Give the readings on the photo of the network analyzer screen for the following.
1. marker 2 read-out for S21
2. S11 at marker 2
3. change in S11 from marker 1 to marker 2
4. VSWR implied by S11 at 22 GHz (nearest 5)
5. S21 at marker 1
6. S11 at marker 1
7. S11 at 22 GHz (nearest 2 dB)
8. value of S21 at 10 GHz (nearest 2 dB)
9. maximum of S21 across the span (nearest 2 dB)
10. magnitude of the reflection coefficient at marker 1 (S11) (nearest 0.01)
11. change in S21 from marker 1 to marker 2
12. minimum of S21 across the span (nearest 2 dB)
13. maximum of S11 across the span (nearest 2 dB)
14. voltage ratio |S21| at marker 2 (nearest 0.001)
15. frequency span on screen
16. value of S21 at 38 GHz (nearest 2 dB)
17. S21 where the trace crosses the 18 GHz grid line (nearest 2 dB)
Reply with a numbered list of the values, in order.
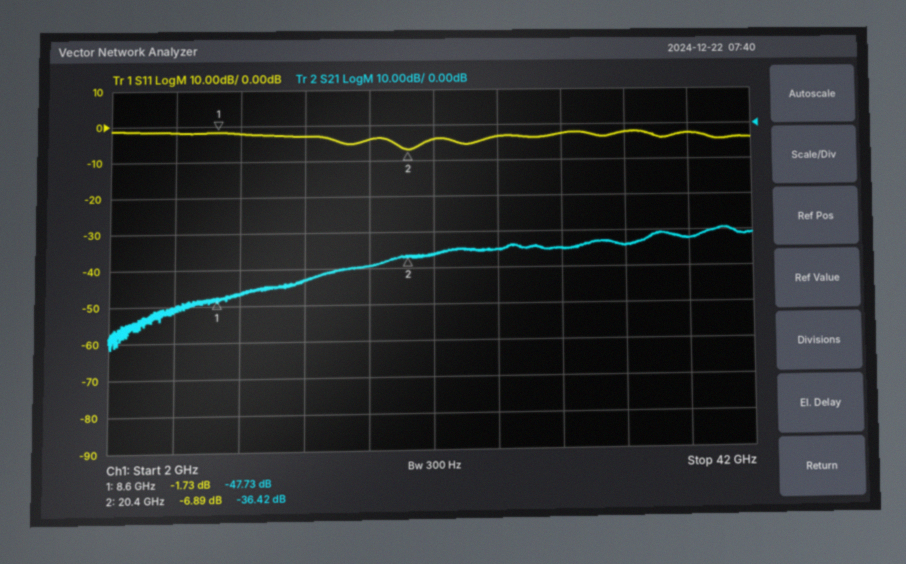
1. -36.42 dB
2. -6.89 dB
3. -5.16 dB
4. 5
5. -47.73 dB
6. -1.73 dB
7. -4 dB
8. -46 dB
9. -30 dB
10. 0.82
11. 11.31 dB
12. -62 dB
13. -2 dB
14. 0.015
15. 40 GHz
16. -32 dB
17. -40 dB
